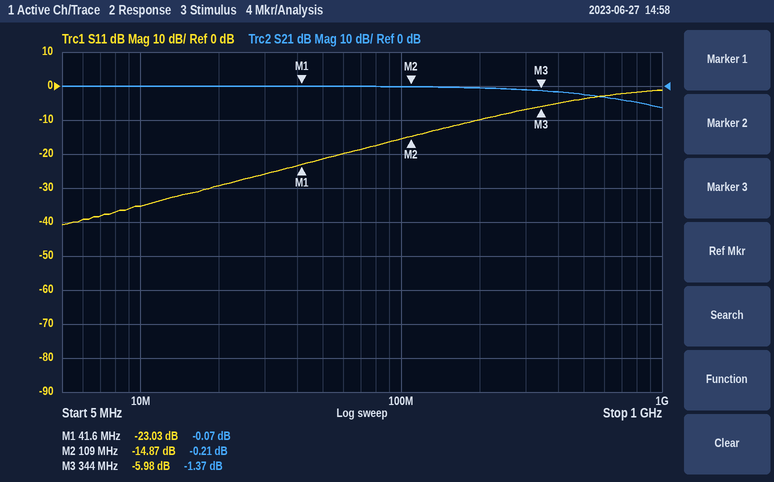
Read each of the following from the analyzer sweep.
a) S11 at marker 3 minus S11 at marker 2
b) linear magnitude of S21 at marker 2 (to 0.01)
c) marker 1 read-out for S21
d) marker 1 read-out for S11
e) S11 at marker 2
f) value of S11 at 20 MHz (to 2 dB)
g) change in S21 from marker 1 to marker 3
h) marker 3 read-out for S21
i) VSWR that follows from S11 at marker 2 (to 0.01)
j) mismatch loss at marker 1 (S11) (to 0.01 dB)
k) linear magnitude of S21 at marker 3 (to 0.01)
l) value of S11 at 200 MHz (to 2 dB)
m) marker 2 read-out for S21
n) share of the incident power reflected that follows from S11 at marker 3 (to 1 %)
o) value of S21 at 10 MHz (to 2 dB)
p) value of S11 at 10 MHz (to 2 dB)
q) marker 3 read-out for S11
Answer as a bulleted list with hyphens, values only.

- 8.89 dB
- 0.98
- -0.07 dB
- -23.03 dB
- -14.87 dB
- -30 dB
- -1.30 dB
- -1.37 dB
- 1.44
- 0.02 dB
- 0.85
- -10 dB
- -0.21 dB
- 25 %
- 0 dB
- -36 dB
- -5.98 dB
